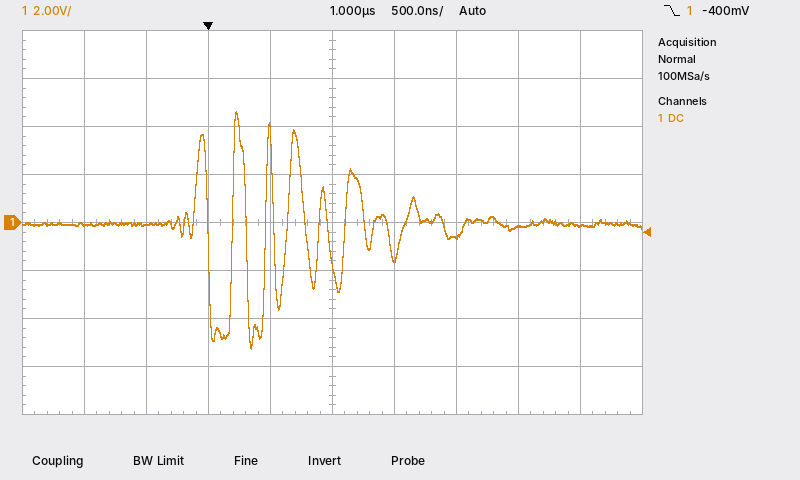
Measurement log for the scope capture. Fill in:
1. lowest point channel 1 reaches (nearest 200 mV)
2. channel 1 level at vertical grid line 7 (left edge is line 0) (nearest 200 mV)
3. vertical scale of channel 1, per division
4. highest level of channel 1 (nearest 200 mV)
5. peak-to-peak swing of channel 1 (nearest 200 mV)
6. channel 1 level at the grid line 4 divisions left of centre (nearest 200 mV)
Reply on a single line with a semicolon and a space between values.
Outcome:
-5.2 V; -600 mV; 2 V; 4.6 V; 9.8 V; 0.0 V
